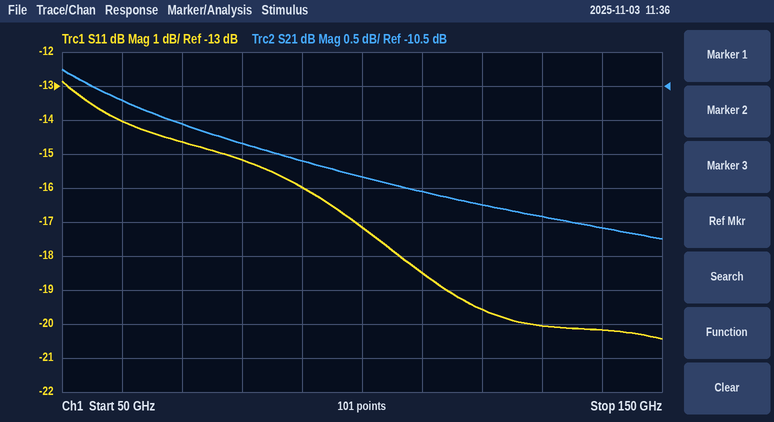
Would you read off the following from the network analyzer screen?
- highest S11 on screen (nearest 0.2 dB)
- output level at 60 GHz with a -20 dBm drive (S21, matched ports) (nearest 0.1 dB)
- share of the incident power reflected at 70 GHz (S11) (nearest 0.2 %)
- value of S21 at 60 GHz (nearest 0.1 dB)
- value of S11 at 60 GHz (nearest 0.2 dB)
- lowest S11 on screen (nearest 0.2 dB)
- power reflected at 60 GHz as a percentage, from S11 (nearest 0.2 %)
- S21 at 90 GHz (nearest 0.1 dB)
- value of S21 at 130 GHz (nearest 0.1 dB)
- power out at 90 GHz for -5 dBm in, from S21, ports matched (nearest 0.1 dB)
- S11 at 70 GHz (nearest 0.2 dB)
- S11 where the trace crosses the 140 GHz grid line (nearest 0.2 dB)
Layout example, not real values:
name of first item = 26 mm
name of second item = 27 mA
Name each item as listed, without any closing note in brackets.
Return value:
highest S11 on screen = -12.8 dB
output level at 60 GHz with a -20 dBm drive (S21, matched ports) = -30.7 dBm
share of the incident power reflected at 70 GHz (S11) = 3.4 %
value of S21 at 60 GHz = -10.7 dB
value of S11 at 60 GHz = -14.0 dB
lowest S11 on screen = -20.4 dB
power reflected at 60 GHz as a percentage, from S11 = 4.0 %
S21 at 90 GHz = -11.6 dB
value of S21 at 130 GHz = -12.4 dB
power out at 90 GHz for -5 dBm in, from S21, ports matched = -16.6 dBm
S11 at 70 GHz = -14.6 dB
S11 where the trace crosses the 140 GHz grid line = -20.2 dB
